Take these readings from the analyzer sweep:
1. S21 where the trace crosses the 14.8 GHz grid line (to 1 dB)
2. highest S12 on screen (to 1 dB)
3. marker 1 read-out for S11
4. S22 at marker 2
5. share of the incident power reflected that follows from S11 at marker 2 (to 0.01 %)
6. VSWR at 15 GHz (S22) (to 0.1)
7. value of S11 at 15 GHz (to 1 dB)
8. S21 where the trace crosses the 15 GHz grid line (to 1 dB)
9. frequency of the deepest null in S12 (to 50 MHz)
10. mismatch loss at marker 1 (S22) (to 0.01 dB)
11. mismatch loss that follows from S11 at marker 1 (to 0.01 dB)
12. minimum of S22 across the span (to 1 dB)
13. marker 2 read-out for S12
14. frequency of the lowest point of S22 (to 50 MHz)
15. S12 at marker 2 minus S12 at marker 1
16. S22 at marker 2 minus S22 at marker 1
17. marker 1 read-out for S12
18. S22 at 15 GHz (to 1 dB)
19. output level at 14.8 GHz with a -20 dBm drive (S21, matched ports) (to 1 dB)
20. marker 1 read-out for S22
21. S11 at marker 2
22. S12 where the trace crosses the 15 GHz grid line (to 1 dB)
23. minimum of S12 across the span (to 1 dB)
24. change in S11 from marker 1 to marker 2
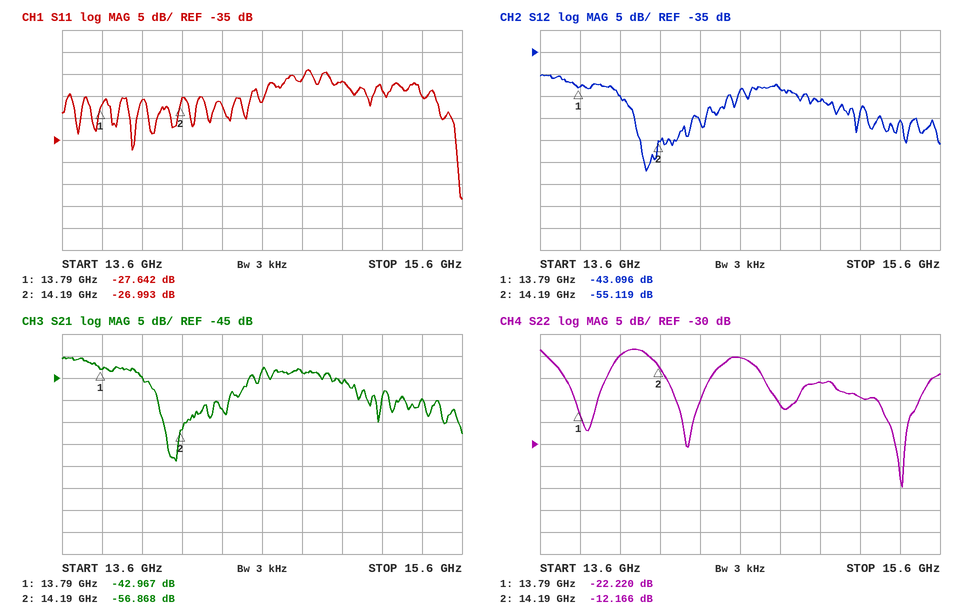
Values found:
-44 dB
-40 dB
-27.642 dB
-12.166 dB
0.20 %
1.4
-22 dB
-46 dB
14.15 GHz
0.03 dB
0.01 dB
-40 dB
-55.119 dB
15.40 GHz
-12.023 dB
10.054 dB
-43.096 dB
-16 dB
-64 dBm
-22.220 dB
-26.993 dB
-46 dB
-62 dB
0.649 dB
